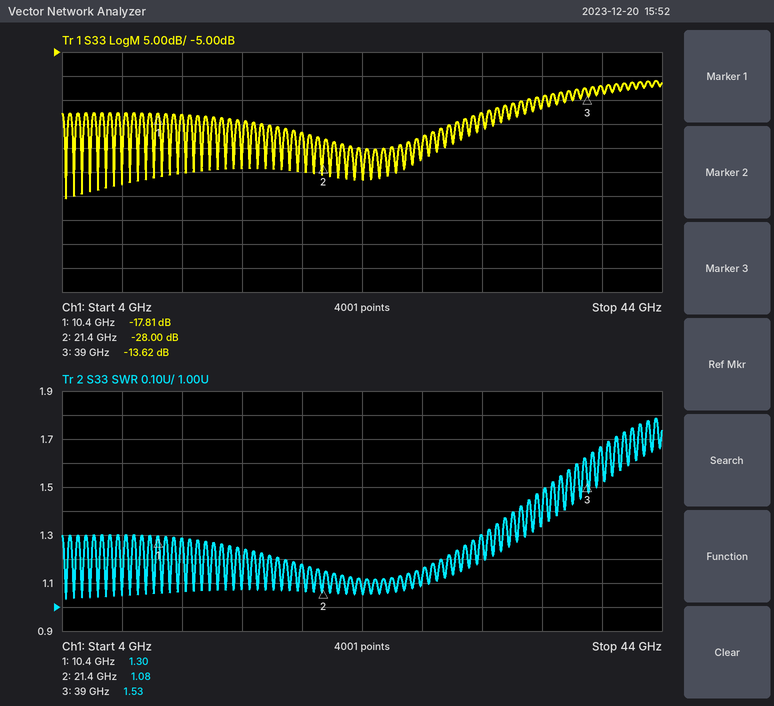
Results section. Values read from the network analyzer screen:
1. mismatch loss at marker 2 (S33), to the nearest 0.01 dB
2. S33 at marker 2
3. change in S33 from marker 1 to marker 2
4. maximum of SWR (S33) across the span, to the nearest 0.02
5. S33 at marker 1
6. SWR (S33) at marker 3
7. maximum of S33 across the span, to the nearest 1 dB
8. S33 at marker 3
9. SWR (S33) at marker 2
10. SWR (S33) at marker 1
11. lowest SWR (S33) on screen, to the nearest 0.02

0.01 dB
-28.00 dB
-10.19 dB
1.78
-17.81 dB
1.53
-11 dB
-13.62 dB
1.08
1.30
1.04
